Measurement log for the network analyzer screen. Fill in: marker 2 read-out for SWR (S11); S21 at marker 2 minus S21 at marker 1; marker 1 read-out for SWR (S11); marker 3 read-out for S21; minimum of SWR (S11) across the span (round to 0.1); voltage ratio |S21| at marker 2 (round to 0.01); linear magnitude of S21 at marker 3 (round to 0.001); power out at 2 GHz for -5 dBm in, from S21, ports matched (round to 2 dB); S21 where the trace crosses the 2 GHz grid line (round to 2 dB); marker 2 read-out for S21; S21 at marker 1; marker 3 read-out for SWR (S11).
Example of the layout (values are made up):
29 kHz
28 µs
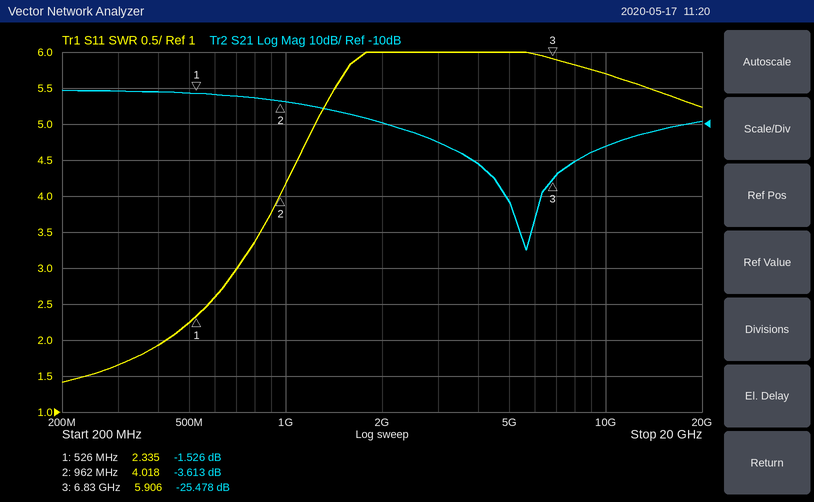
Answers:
4.018
-2.087 dB
2.335
-25.478 dB
1.4
0.66
0.053
-14 dBm
-10 dB
-3.613 dB
-1.526 dB
5.906
